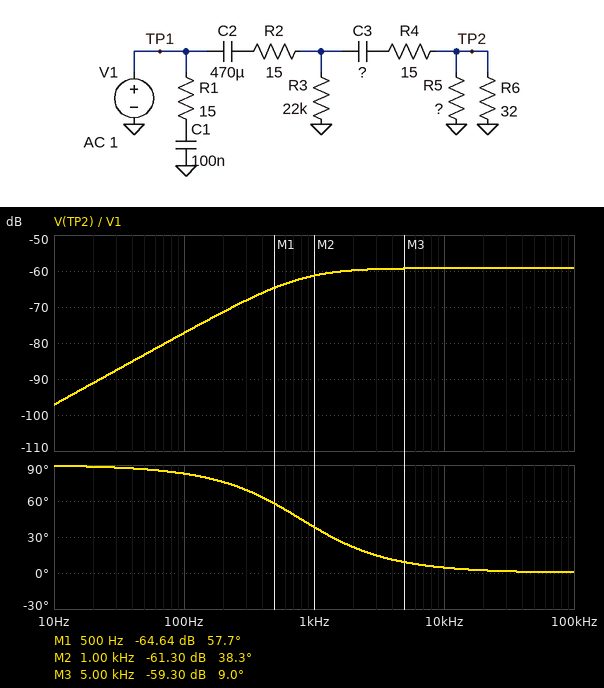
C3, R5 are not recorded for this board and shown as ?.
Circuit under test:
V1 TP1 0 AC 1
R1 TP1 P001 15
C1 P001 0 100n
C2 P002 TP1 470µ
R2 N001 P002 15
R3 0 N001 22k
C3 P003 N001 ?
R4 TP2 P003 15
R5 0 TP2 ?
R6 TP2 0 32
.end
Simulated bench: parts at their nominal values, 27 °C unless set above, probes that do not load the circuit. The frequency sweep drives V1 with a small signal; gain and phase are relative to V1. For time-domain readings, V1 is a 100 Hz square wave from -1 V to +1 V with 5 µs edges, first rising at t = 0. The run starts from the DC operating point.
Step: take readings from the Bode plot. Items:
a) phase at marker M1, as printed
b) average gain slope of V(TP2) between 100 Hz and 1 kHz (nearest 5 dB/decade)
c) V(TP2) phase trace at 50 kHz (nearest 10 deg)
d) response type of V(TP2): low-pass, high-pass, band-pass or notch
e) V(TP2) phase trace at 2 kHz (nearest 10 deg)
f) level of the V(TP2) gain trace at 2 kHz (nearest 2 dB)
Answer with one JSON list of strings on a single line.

["57.7 deg", "15 dB/decade", "0 deg", "high-pass", "20 deg", "-60 dB"]
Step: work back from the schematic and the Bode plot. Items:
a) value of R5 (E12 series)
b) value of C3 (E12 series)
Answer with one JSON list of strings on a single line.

["0.033 Ω", "6.8 µF"]
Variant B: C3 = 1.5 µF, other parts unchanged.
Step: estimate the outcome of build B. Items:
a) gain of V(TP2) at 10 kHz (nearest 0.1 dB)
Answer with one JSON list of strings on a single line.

["-59.7 dB"]
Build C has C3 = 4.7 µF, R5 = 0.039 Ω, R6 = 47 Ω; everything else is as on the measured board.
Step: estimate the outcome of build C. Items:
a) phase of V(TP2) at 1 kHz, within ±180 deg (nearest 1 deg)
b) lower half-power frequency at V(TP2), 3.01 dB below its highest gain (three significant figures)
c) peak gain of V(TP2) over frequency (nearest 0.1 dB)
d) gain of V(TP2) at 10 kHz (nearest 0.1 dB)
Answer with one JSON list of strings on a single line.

["49 deg", "1.14 kHz", "-57.7 dB", "-57.8 dB"]
